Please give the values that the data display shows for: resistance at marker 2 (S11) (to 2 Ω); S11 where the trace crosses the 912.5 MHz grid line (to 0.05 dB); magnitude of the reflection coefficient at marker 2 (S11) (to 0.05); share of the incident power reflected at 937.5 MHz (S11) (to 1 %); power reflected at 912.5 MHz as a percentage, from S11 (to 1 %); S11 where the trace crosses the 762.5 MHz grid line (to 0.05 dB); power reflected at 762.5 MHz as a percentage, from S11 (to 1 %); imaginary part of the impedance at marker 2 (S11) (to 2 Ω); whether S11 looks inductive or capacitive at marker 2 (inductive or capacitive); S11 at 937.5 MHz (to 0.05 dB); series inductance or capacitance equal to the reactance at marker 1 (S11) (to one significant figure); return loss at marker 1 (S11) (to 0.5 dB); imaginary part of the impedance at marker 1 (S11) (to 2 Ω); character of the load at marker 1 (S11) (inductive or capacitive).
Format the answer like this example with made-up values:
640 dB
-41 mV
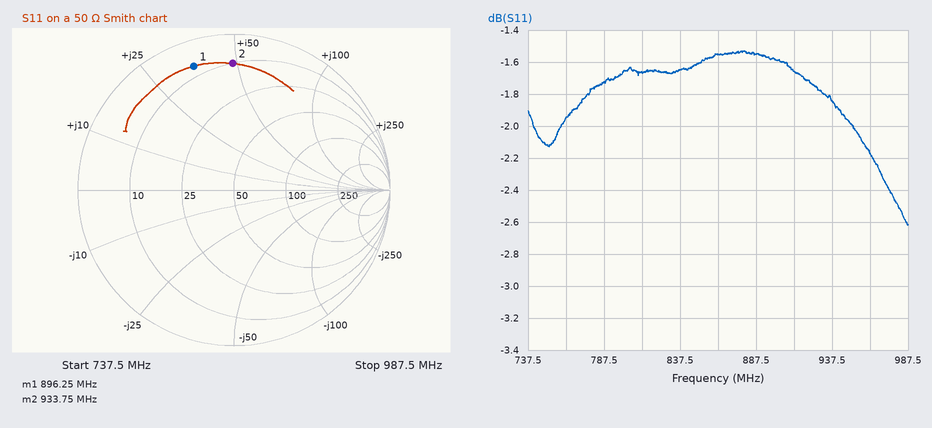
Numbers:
10 Ω
-1.65 dB
0.80
65 %
68 %
-1.95 dB
64 %
+48 Ω
inductive
-1.85 dB
6 nH
1.5 dB
+36 Ω
inductive
